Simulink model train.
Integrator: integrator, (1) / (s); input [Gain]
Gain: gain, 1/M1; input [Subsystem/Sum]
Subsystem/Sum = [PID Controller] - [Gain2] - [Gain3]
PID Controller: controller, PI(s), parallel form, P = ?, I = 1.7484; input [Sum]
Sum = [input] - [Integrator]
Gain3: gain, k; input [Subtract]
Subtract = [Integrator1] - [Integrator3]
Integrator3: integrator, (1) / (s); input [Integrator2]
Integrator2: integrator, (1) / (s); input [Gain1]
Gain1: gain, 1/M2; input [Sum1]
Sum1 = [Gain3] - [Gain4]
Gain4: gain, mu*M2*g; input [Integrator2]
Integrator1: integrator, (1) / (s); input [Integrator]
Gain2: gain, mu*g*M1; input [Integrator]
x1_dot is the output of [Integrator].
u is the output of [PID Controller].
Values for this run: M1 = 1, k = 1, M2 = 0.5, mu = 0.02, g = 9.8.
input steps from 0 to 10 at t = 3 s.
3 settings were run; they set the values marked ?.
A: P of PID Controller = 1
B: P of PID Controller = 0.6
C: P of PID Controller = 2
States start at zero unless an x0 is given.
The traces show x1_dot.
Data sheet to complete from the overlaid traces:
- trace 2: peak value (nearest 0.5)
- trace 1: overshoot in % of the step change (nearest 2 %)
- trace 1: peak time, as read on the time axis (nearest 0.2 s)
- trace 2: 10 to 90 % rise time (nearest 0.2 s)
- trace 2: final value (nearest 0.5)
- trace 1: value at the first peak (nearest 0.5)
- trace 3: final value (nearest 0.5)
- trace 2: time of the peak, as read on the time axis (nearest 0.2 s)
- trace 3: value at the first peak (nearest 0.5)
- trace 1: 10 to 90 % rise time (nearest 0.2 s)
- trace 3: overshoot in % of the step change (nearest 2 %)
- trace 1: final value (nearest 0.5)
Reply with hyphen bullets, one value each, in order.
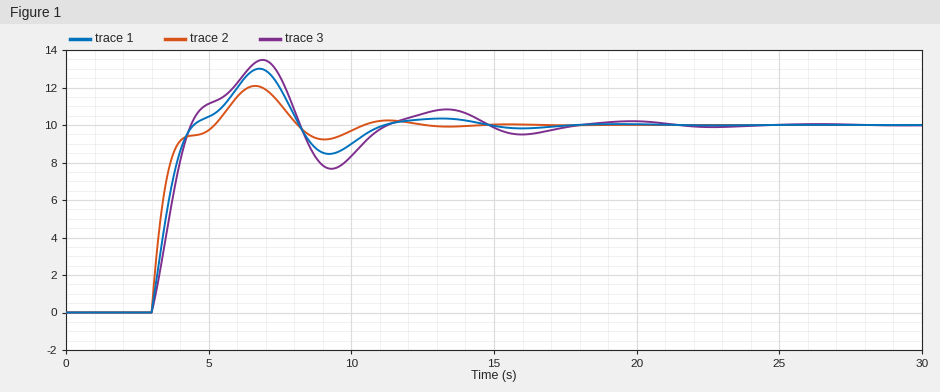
- 12.0
- 30 %
- 6.8 s
- 0.8 s
- 10.0
- 13.0
- 10.0
- 6.6 s
- 13.5
- 1.0 s
- 34 %
- 10.0
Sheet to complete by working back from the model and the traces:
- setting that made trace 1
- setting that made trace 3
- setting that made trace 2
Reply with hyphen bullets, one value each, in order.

- A
- B
- C
